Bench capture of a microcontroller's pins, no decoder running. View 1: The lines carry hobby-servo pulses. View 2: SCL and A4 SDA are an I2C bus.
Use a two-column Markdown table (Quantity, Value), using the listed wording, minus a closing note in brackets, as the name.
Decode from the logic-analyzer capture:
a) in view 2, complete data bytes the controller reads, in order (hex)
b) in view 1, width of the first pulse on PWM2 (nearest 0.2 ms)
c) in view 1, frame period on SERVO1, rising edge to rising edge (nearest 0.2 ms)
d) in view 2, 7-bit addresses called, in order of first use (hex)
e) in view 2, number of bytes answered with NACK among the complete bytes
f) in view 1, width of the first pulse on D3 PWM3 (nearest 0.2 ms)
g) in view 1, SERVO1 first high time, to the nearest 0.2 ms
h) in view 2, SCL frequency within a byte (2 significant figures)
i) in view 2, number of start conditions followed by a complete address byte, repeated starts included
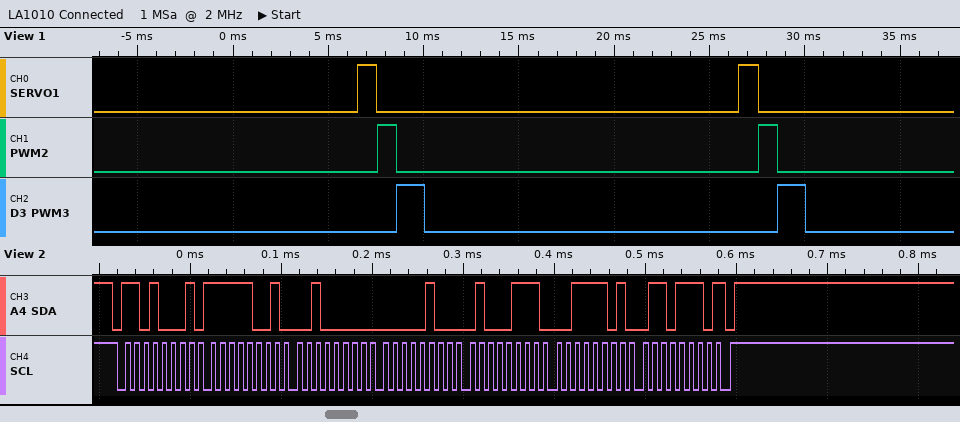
| Quantity | Value |
|---|---|
| in view 2, complete data bytes the controller reads, in order | F9 20 04 47 3D 6E |
| in view 1, width of the first pulse on PWM2 | 1.0 ms |
| in view 1, frame period on SERVO1, rising edge to rising edge | 20.0 ms |
| in view 2, 7-bit addresses called, in order of first use | 0x68 |
| in view 2, number of bytes answered with NACK among the complete bytes | 1 |
| in view 1, width of the first pulse on D3 PWM3 | 1.4 ms |
| in view 1, SERVO1 first high time, to the nearest 0.2 ms | 1.0 ms |
| in view 2, SCL frequency within a byte | 100 kHz |
| in view 2, number of start conditions followed by a complete address byte, repeated starts included | 1 |
